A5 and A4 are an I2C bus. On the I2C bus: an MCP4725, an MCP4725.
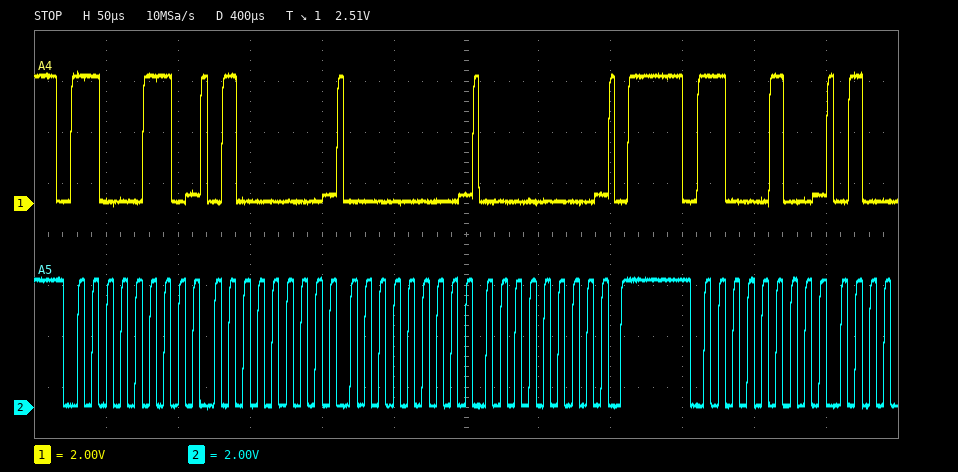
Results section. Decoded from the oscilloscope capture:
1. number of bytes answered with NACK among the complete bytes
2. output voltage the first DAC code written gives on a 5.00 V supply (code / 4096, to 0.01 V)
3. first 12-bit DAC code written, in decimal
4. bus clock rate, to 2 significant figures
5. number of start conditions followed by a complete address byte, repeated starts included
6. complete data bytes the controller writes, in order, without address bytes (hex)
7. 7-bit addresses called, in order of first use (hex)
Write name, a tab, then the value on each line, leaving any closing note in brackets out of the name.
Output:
number of bytes answered with NACK among the complete bytes	0
output voltage the first DAC code written gives on a 5.00 V supply	0.00 V
first 12-bit DAC code written, in decimal	0
bus clock rate, to 2 significant figures	100 kHz
number of start conditions followed by a complete address byte, repeated starts included	2
complete data bytes the controller writes, in order, without address bytes	40 00 00
7-bit addresses called, in order of first use	0x63 0x62
